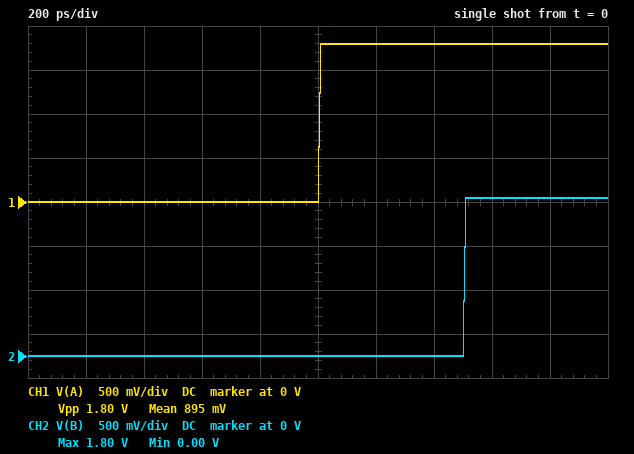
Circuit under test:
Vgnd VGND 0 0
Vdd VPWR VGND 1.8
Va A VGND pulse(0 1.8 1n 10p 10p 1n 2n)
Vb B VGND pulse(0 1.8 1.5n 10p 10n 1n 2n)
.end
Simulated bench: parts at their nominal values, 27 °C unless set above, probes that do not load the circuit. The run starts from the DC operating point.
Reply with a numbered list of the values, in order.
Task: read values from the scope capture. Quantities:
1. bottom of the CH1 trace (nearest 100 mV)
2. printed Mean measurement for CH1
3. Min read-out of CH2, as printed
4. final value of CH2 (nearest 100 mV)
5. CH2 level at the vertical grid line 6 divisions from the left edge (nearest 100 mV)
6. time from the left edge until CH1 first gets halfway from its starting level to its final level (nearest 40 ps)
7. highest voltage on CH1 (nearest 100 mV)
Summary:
1. 0 V
2. 895 mV
3. 0.00 V
4. 1.8 V
5. 0 V
6. 1.00 ns
7. 1.8 V
